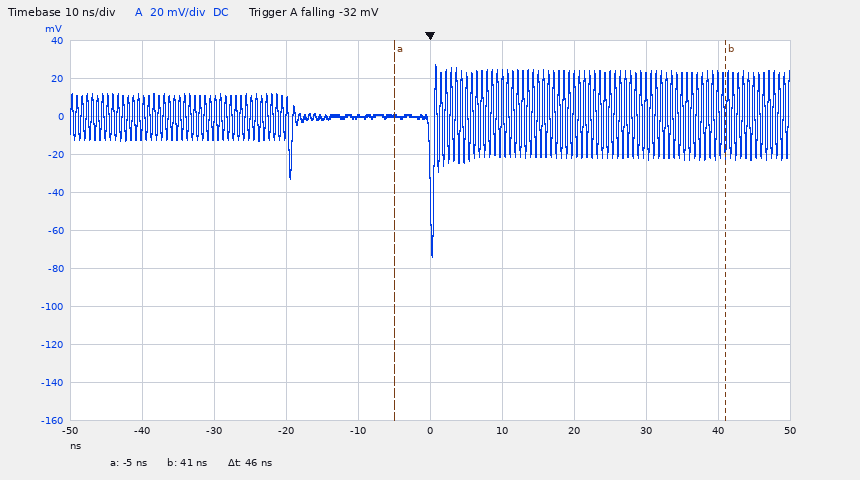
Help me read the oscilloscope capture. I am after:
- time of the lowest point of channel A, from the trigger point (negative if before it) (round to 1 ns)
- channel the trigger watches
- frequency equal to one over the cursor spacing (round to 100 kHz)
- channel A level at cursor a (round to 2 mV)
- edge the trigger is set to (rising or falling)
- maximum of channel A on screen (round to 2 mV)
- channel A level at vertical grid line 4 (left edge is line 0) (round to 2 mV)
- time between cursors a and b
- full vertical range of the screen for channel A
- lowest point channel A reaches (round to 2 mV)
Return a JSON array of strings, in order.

["0 ns", "channel A", "21.7 MHz", "0 mV", "falling", "28 mV", "0 mV", "46 ns", "200 mV", "-74 mV"]
